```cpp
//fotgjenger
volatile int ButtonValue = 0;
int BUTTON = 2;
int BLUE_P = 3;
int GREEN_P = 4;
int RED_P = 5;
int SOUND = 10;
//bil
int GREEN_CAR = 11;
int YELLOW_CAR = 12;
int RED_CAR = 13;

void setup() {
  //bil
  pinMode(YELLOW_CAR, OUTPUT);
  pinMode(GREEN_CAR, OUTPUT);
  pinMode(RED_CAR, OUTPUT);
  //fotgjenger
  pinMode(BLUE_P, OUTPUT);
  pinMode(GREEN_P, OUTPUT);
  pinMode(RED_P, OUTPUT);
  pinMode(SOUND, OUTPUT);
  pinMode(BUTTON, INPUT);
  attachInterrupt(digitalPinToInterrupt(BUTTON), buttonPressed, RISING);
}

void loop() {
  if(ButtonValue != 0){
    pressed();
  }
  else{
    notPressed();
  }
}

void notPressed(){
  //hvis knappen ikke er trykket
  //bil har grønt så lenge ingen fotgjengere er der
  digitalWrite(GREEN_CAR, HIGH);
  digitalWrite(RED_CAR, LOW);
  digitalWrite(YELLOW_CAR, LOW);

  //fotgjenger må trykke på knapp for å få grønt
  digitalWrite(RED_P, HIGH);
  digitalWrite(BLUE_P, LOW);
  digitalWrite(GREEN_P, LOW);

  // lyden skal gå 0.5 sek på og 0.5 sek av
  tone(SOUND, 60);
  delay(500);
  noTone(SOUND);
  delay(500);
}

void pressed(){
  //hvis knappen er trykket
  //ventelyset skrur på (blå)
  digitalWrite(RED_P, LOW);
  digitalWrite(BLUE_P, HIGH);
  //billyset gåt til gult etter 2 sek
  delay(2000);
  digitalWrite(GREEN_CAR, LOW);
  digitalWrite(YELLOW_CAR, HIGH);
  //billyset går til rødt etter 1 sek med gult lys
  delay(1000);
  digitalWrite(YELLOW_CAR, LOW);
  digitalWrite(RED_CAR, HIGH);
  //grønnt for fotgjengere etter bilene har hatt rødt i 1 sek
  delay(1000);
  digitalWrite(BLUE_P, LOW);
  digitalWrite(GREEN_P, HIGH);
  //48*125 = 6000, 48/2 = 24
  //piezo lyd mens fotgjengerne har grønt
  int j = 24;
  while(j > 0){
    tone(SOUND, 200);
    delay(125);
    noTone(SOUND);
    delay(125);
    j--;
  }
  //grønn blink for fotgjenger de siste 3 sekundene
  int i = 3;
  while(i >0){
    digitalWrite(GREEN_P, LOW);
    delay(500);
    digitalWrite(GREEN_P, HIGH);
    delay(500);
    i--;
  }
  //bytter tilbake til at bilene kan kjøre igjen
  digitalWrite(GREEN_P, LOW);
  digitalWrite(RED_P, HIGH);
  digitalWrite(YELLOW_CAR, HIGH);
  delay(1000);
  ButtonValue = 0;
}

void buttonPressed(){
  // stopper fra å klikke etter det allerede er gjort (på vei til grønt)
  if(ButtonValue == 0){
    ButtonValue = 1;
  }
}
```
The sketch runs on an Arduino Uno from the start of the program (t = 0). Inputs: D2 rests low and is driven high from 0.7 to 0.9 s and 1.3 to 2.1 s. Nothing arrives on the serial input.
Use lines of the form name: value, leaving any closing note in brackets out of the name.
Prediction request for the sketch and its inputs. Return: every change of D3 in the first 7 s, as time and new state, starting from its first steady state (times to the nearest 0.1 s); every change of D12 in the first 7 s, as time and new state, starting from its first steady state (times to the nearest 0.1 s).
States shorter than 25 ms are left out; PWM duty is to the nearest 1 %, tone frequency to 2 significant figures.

every change of D3 in the first 7 s, as time and new state, starting from its first steady state: 0 s low; 1 s high; 5 s low
every change of D12 in the first 7 s, as time and new state, starting from its first steady state: 0 s low; 3 s high; 4 s low
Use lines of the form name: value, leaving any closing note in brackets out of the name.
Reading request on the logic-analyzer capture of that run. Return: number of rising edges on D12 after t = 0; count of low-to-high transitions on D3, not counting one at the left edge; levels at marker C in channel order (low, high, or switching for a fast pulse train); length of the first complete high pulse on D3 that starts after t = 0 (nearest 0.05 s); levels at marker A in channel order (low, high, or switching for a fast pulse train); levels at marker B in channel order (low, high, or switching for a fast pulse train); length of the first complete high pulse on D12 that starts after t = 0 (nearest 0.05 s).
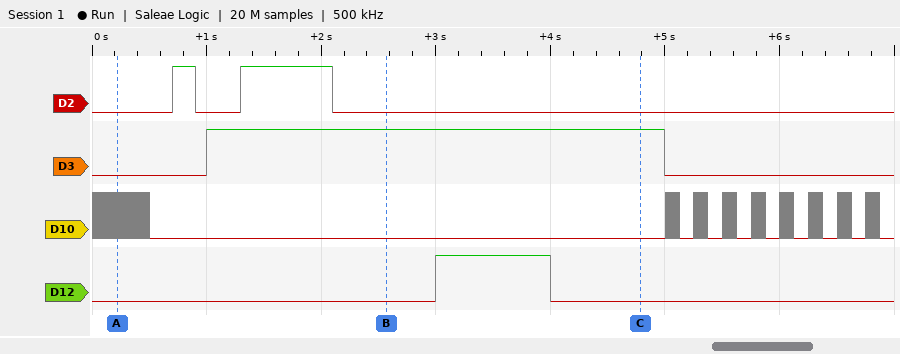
number of rising edges on D12 after t = 0: 1
count of low-to-high transitions on D3, not counting one at the left edge: 1
levels at marker C in channel order: D2 low, D3 high, D10 low, D12 low
length of the first complete high pulse on D3 that starts after t = 0: 4.00 s
levels at marker A in channel order: D2 low, D3 low, D10 switching, D12 low
levels at marker B in channel order: D2 low, D3 high, D10 low, D12 low
length of the first complete high pulse on D12 that starts after t = 0: 1.00 s
